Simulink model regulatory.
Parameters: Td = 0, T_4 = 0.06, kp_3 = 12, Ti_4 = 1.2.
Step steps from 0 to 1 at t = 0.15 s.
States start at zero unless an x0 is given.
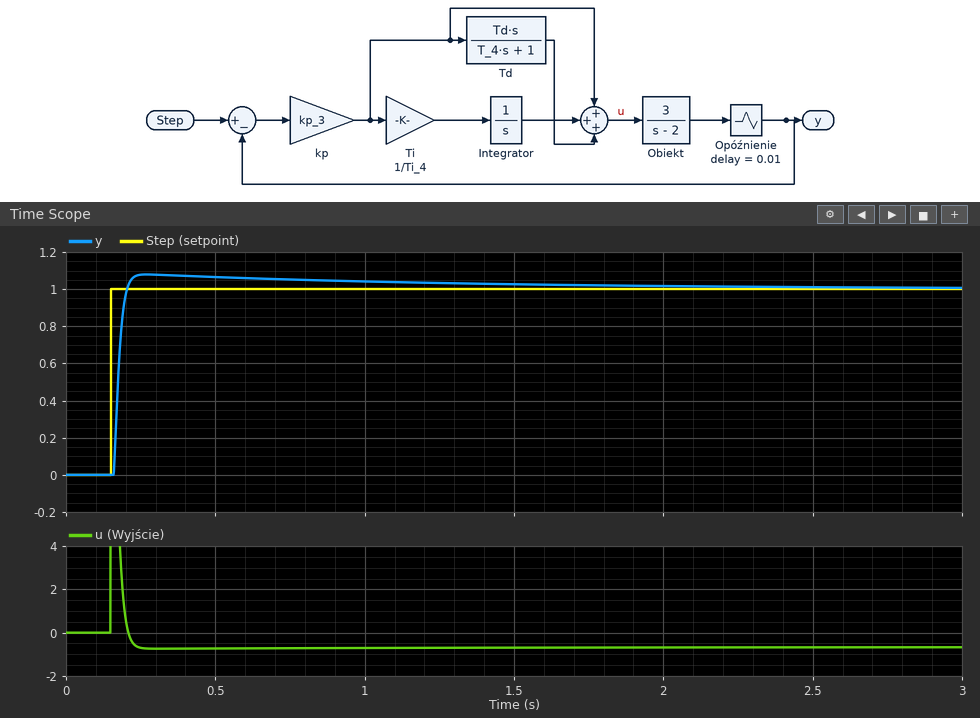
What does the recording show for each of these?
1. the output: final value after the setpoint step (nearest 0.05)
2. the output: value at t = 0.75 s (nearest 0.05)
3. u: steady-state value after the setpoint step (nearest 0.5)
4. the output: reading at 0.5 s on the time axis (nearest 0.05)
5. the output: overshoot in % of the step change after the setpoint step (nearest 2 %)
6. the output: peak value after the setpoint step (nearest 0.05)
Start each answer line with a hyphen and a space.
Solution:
- 1.00
- 1.05
- -0.5
- 1.05
- 8 %
- 1.10
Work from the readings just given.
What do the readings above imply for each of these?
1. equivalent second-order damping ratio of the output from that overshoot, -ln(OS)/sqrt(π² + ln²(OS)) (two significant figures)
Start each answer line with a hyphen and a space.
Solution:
- 0.63
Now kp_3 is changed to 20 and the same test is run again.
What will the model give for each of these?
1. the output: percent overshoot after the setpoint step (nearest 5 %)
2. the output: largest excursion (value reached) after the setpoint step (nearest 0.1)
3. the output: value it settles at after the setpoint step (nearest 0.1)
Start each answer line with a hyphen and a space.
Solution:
- 15 %
- 1.2
- 1.0
